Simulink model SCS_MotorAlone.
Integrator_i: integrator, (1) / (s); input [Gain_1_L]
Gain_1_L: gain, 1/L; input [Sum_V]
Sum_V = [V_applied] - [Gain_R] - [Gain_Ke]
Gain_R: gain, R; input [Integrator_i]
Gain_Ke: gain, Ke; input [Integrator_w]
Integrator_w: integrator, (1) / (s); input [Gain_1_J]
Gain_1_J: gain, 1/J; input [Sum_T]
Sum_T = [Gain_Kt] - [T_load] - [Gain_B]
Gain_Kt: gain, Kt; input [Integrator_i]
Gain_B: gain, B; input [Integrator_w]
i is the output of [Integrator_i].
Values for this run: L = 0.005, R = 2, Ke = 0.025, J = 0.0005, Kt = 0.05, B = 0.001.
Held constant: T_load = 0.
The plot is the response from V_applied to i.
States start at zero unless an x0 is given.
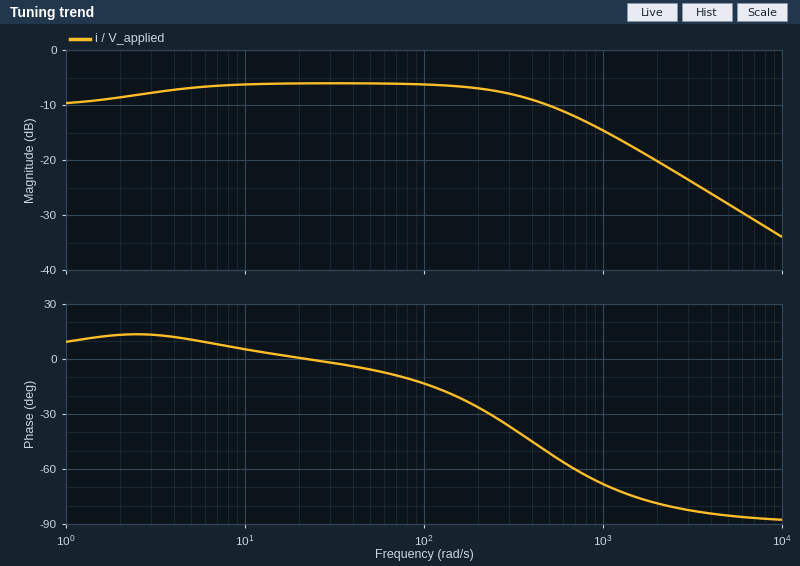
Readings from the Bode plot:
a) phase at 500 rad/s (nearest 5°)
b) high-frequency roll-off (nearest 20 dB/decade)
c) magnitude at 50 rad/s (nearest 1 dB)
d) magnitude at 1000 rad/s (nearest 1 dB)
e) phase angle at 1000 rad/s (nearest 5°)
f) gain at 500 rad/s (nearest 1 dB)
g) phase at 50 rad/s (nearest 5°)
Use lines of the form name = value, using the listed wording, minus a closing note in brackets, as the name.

phase at 500 rad/s = -50°
high-frequency roll-off = -20 dB/decade
magnitude at 50 rad/s = -6 dB
magnitude at 1000 rad/s = -15 dB
phase angle at 1000 rad/s = -70°
gain at 500 rad/s = -10 dB
phase at 50 rad/s = -5°
